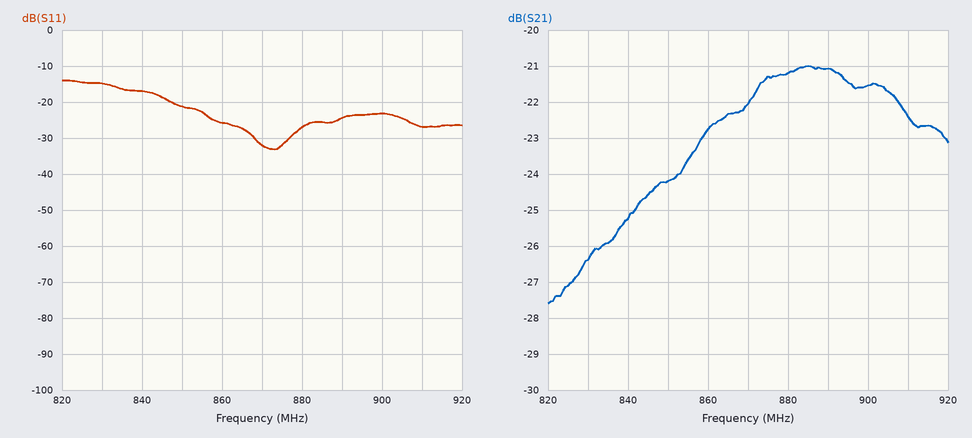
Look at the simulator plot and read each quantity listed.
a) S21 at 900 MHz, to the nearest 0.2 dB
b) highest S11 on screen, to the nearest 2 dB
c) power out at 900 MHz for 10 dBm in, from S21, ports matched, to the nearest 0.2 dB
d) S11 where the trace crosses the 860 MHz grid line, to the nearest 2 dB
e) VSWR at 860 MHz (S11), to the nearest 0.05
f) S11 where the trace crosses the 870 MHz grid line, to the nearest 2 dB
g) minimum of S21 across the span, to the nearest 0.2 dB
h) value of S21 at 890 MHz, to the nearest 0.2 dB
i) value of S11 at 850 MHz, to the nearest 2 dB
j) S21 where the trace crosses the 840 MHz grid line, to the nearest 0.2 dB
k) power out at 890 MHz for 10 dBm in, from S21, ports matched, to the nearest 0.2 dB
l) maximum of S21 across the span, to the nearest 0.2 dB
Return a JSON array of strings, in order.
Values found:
["-21.6 dB", "-14 dB", "-11.6 dBm", "-26 dB", "1.10", "-32 dB", "-27.6 dB", "-21.0 dB", "-22 dB", "-25.2 dB", "-11.0 dBm", "-21.0 dB"]
